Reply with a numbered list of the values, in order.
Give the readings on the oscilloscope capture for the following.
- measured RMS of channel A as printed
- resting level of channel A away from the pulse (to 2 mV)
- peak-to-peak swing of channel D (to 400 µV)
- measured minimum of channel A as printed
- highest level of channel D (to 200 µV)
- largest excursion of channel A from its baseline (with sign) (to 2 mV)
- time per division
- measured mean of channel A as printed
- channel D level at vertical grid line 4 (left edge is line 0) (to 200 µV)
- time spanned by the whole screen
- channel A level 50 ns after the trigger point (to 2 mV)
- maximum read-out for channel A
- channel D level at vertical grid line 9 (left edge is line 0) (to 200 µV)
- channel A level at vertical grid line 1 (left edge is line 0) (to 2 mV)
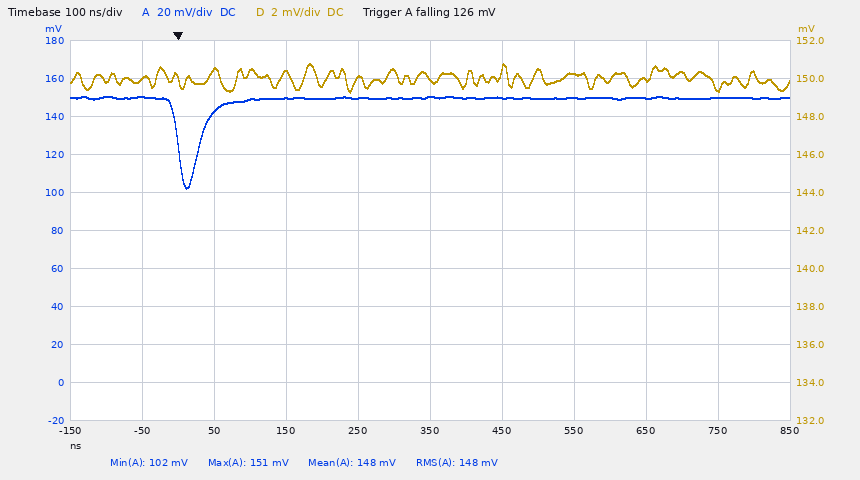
1. 148 mV
2. 150 mV
3. 1.6 mV
4. 102 mV
5. 150.8 mV
6. -48 mV
7. 100 ns
8. 148 mV
9. 150.0 mV
10. 1 µs
11. 142 mV
12. 151 mV
13. 149.4 mV
14. 150 mV
